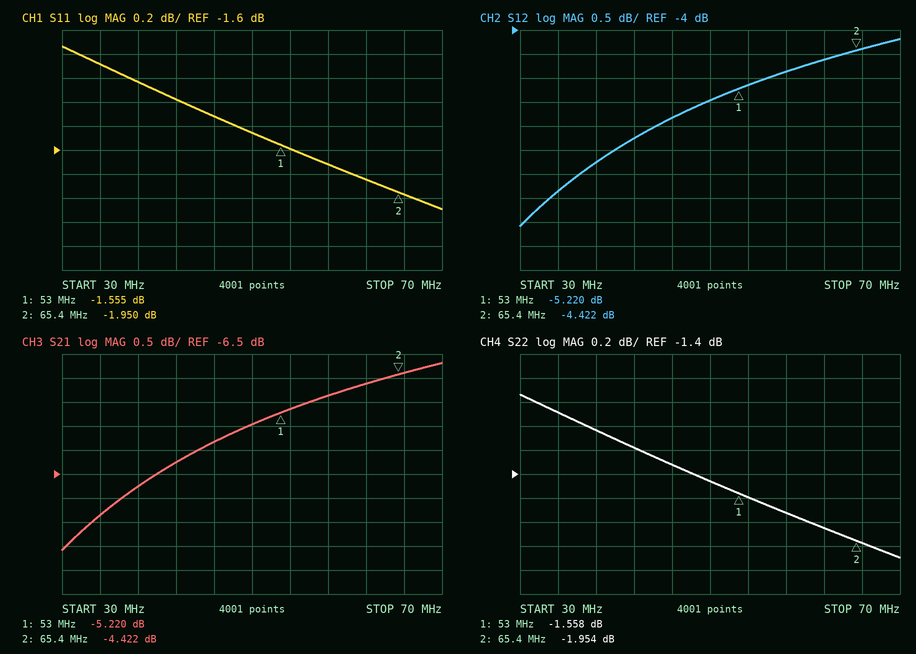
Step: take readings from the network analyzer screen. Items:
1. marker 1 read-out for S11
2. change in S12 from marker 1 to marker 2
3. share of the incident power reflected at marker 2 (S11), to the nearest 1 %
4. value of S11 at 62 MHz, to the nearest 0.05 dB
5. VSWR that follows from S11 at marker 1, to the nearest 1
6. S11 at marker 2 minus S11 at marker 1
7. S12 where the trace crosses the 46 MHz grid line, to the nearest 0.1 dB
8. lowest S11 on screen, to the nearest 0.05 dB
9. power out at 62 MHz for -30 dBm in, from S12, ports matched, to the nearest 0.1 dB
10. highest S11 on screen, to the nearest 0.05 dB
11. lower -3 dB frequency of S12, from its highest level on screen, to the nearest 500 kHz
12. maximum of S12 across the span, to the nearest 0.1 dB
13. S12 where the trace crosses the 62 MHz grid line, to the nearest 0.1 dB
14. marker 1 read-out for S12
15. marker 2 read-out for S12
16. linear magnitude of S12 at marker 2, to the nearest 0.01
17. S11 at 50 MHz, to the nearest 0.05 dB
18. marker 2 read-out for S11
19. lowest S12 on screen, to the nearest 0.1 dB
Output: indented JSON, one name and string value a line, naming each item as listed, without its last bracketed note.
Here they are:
{
  "marker 1 read-out for S11": "-1.555 dB",
  "change in S12 from marker 1 to marker 2": "0.798 dB",
  "share of the incident power reflected at marker 2 (S11), to the nearest 1 %": "64 %",
  "value of S11 at 62 MHz, to the nearest 0.05 dB": "-1.85 dB",
  "VSWR that follows from S11 at marker 1, to the nearest 1": "11",
  "S11 at marker 2 minus S11 at marker 1": "-0.395 dB",
  "S12 where the trace crosses the 46 MHz grid line, to the nearest 0.1 dB": "-5.8 dB",
  "lowest S11 on screen, to the nearest 0.05 dB": "-2.10 dB",
  "power out at 62 MHz for -30 dBm in, from S12, ports matched, to the nearest 0.1 dB": "-34.6 dBm",
  "highest S11 on screen, to the nearest 0.05 dB": "-0.75 dB",
  "lower -3 dB frequency of S12, from its highest level on screen, to the nearest 500 kHz": "35.0 MHz",
  "maximum of S12 across the span, to the nearest 0.1 dB": "-4.2 dB",
  "S12 where the trace crosses the 62 MHz grid line, to the nearest 0.1 dB": "-4.6 dB",
  "marker 1 read-out for S12": "-5.220 dB",
  "marker 2 read-out for S12": "-4.422 dB",
  "linear magnitude of S12 at marker 2, to the nearest 0.01": "0.60",
  "S11 at 50 MHz, to the nearest 0.05 dB": "-1.45 dB",
  "marker 2 read-out for S11": "-1.950 dB",
  "lowest S12 on screen, to the nearest 0.1 dB": "-8.1 dB"
}
